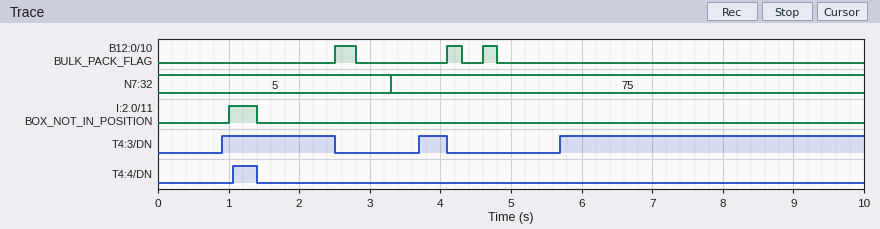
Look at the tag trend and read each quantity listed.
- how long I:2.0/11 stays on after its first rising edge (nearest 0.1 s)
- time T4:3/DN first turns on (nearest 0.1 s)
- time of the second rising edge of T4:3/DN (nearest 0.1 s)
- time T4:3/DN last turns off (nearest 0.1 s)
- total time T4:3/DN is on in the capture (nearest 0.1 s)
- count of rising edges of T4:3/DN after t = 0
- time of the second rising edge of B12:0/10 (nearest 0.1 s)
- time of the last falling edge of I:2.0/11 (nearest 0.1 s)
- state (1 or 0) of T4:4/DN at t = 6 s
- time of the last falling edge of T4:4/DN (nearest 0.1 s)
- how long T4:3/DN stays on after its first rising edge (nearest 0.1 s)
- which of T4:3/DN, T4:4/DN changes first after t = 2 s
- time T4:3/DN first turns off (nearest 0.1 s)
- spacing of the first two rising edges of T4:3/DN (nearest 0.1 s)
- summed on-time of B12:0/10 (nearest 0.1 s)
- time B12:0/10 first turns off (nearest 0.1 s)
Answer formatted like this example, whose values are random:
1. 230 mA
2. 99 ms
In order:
1. 0.4 s
2. 0.9 s
3. 3.7 s
4. 4.1 s
5. 6.3 s
6. 3
7. 4.1 s
8. 1.4 s
9. 0
10. 1.4 s
11. 1.6 s
12. T4:3/DN
13. 2.5 s
14. 2.8 s
15. 0.7 s
16. 2.8 s
